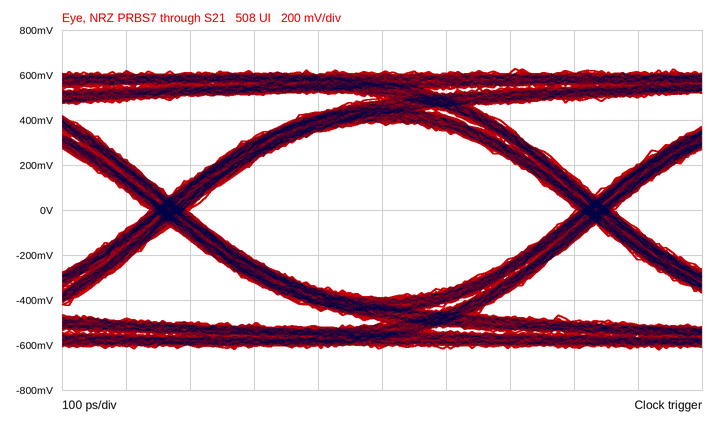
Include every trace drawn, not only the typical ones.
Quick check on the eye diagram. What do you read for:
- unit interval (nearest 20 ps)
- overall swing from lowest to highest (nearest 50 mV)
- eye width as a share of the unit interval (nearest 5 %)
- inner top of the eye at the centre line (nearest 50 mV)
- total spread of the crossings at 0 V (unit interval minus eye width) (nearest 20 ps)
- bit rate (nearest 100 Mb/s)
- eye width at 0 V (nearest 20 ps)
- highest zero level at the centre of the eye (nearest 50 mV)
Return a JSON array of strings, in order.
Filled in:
["660 ps", "1.25 V", "90 %", "400 mV", "60 ps", "1.5 Gb/s", "600 ps", "-400 mV"]
